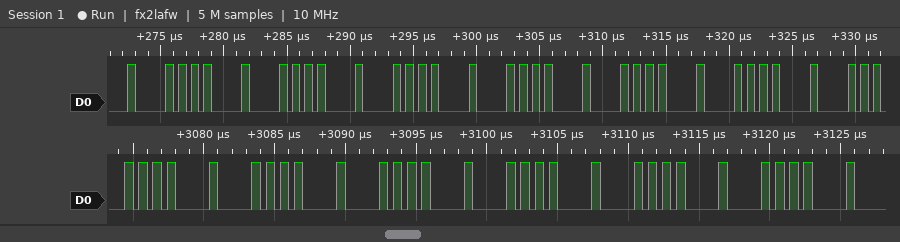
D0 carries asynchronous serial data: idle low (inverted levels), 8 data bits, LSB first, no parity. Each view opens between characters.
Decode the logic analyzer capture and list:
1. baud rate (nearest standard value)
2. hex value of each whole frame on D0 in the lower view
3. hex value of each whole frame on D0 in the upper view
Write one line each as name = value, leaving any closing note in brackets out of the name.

baud rate = 2000000 baud
hex value of each whole frame on D0 in the lower view = D5, 5F, 7D, D5, 5F, 7D, D5, 5F, 7D
hex value of each whole frame on D0 in the upper view = 5F, 7D, D5, 5F, 7D, D5, 5F, 7D, D5, 5F
